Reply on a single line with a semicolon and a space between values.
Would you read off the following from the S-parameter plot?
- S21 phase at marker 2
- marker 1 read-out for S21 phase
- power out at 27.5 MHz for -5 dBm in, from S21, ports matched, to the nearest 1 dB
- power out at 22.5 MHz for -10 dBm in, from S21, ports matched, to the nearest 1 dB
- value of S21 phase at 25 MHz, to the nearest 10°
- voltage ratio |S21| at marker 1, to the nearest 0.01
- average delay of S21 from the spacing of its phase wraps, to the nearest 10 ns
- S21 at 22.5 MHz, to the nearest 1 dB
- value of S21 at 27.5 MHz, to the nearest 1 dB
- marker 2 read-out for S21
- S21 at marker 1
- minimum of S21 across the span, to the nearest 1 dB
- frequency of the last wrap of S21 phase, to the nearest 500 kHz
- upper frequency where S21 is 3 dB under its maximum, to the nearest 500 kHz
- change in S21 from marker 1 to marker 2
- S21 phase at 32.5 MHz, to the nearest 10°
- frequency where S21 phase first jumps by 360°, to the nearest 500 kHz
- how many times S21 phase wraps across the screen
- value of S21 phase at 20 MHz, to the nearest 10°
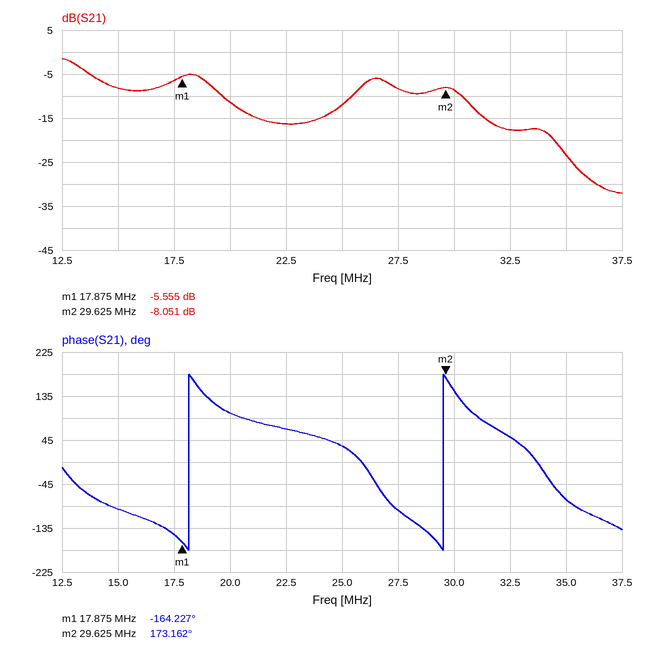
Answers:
173.162°; -164.227°; -13 dBm; -26 dBm; 30°; 0.53; 90 ns; -16 dB; -8 dB; -8.051 dB; -5.555 dB; -32 dB; 29.5 MHz; 13.5 MHz; -2.496 dB; 50°; 18.0 MHz; 2; 100°
